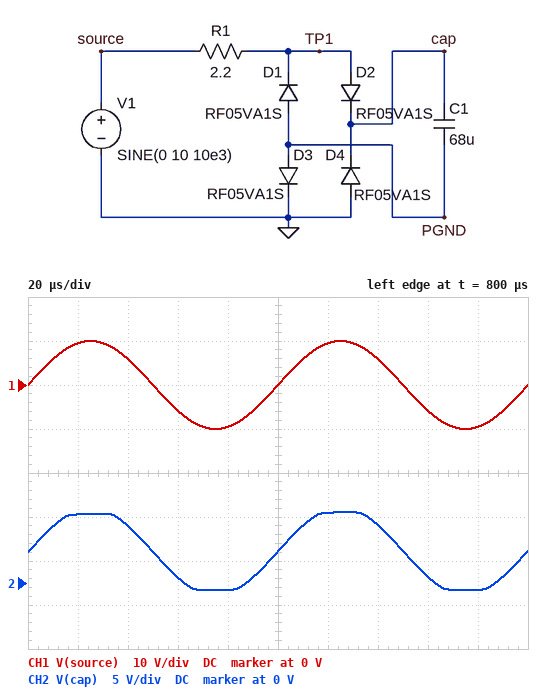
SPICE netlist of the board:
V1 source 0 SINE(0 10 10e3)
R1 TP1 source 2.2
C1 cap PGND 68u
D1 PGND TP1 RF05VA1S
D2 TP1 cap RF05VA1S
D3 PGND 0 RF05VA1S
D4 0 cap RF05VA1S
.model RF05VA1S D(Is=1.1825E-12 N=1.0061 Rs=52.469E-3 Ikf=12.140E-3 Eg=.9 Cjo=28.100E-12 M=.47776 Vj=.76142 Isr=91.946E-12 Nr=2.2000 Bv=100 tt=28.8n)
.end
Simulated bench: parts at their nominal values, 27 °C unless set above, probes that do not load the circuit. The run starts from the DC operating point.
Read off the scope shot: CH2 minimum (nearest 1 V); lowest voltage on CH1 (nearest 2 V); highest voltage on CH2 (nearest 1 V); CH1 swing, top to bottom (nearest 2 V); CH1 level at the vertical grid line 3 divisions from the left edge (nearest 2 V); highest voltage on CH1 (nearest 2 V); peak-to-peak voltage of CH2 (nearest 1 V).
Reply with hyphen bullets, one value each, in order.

- -1 V
- -10 V
- 8 V
- 20 V
- -6 V
- 10 V
- 9 V
